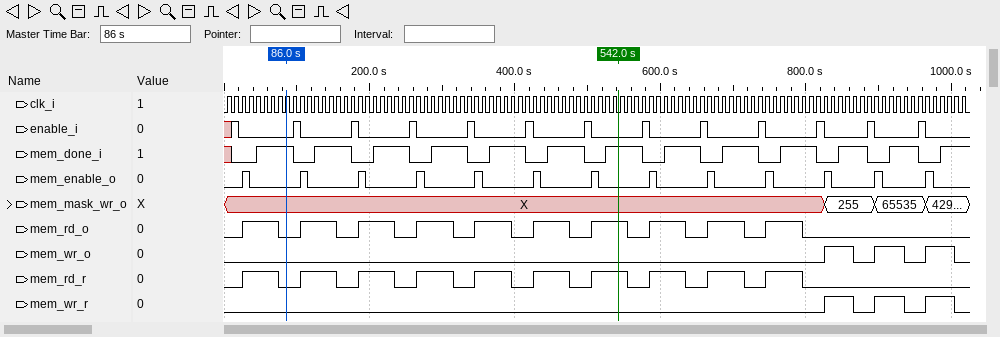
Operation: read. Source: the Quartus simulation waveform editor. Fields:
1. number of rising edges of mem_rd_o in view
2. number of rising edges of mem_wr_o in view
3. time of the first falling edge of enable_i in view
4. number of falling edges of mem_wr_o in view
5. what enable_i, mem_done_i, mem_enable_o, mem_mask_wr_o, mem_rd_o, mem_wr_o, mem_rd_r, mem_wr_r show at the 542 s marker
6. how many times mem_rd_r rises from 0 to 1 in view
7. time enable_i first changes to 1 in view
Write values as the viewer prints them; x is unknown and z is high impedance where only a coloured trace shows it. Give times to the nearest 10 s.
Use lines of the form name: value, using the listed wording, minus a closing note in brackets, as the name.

number of rising edges of mem_rd_o in view: 10
number of rising edges of mem_wr_o in view: 3
time of the first falling edge of enable_i in view: 20 s
number of falling edges of mem_wr_o in view: 3
what enable_i, mem_done_i, mem_enable_o, mem_mask_wr_o, mem_rd_o, mem_wr_o, mem_rd_r, mem_wr_r show at the 542 s marker: enable_i=0, mem_done_i=1, mem_enable_o=0, mem_mask_wr_o=X, mem_rd_o=1, mem_wr_o=0, mem_rd_r=1, mem_wr_r=0
how many times mem_rd_r rises from 0 to 1 in view: 10
time enable_i first changes to 1 in view: 10 s
